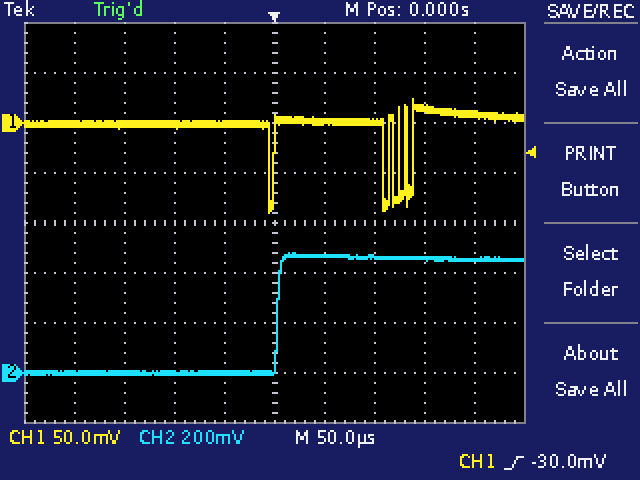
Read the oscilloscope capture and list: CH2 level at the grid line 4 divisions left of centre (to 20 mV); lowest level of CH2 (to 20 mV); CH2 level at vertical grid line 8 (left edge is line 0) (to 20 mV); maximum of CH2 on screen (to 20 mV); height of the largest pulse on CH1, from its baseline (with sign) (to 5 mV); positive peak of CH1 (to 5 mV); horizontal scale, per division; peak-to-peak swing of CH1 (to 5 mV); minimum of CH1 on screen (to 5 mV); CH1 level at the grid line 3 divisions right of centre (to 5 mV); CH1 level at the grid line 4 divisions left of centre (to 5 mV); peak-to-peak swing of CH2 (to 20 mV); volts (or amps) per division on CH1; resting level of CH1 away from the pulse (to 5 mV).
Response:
0 mV
0 mV
460 mV
480 mV
-90 mV
25 mV
50 µs
115 mV
-90 mV
15 mV
0 mV
480 mV
50 mV
0 mV
